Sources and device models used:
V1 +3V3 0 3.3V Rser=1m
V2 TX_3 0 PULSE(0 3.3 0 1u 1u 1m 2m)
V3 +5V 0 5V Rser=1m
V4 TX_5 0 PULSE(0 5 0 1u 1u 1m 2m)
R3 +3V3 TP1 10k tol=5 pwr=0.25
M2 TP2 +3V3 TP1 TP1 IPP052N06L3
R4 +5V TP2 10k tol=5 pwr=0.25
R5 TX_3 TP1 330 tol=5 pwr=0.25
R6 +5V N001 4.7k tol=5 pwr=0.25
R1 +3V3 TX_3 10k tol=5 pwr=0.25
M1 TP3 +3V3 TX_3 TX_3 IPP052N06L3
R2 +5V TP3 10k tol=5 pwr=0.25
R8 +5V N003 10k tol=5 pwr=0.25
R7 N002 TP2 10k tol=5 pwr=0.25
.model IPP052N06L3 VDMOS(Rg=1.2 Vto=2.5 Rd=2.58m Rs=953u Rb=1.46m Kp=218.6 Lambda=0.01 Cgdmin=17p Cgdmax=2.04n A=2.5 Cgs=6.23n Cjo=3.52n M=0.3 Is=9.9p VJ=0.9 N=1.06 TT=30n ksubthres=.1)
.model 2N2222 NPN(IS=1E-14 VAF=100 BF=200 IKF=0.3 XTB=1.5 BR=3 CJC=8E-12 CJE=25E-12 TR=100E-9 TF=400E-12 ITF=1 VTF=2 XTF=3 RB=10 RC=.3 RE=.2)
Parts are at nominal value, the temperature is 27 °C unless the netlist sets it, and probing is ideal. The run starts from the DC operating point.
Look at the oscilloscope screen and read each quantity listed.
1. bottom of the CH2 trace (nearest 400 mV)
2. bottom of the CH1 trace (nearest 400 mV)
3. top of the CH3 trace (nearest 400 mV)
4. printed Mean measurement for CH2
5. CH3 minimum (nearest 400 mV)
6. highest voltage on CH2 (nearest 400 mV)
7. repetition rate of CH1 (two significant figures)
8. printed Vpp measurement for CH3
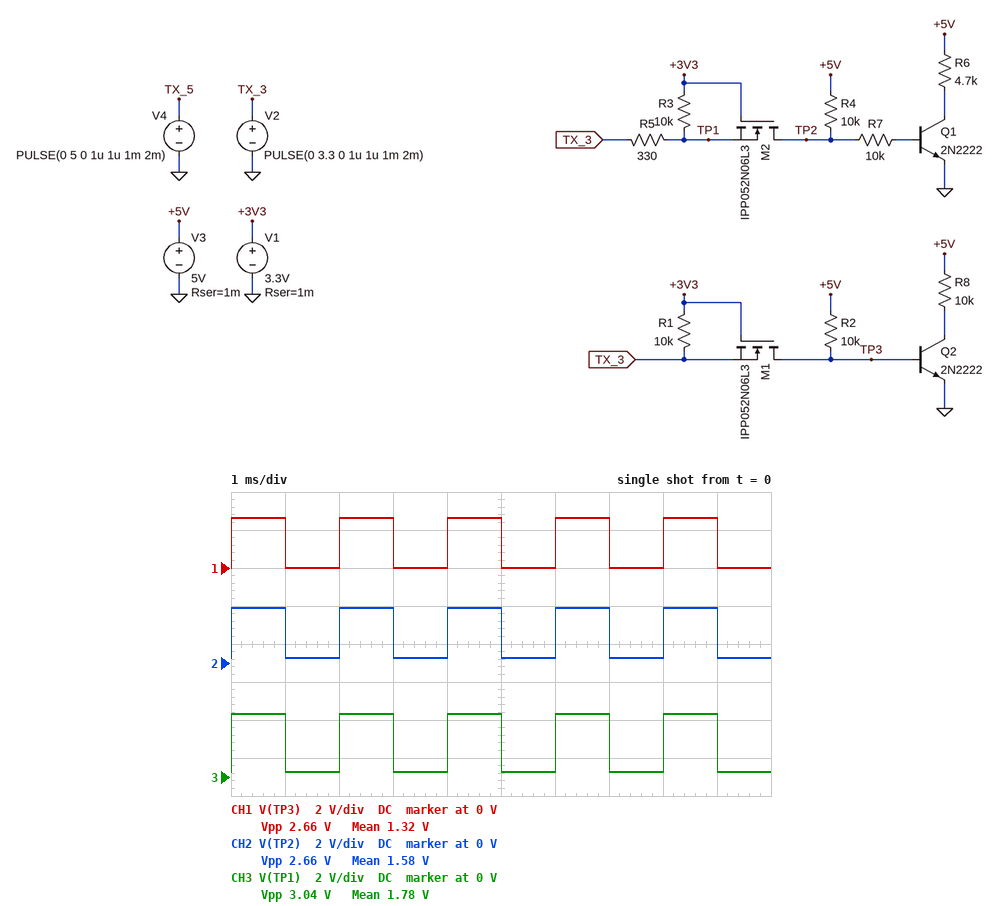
400 mV
0 V
3.2 V
1.58 V
400 mV
2.8 V
500 Hz
3.04 V
